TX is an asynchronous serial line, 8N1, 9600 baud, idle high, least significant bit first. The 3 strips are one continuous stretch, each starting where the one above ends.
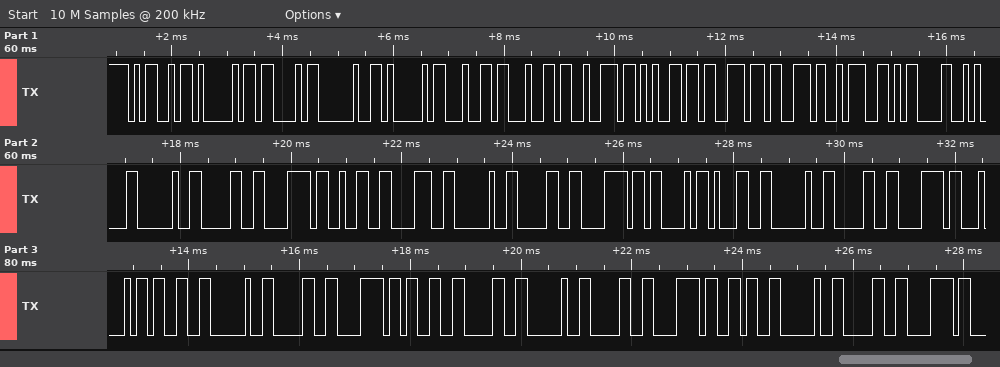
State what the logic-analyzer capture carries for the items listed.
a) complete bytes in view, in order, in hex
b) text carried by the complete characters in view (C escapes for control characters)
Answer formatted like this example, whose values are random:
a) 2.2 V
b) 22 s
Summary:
a) 4D 41 43 20 41 64 64 72 65 73 73 3A 0D 0A 20 30 78 32 38 20 30 78 43 31 20 30 78 44 33 20 30 78 33 30 20 30 78 36 20 30 78
b) "MAC Address:\r\n 0x28 0xC1 0xD3 0x30 0x6 0x"
